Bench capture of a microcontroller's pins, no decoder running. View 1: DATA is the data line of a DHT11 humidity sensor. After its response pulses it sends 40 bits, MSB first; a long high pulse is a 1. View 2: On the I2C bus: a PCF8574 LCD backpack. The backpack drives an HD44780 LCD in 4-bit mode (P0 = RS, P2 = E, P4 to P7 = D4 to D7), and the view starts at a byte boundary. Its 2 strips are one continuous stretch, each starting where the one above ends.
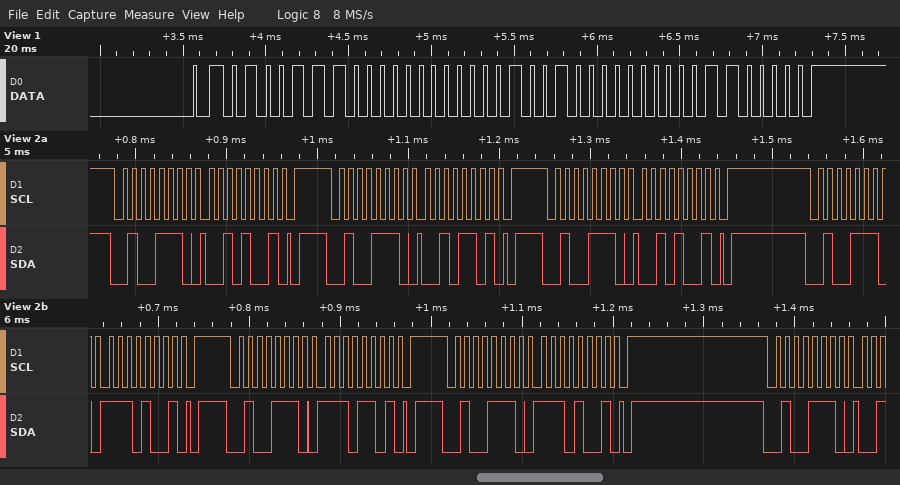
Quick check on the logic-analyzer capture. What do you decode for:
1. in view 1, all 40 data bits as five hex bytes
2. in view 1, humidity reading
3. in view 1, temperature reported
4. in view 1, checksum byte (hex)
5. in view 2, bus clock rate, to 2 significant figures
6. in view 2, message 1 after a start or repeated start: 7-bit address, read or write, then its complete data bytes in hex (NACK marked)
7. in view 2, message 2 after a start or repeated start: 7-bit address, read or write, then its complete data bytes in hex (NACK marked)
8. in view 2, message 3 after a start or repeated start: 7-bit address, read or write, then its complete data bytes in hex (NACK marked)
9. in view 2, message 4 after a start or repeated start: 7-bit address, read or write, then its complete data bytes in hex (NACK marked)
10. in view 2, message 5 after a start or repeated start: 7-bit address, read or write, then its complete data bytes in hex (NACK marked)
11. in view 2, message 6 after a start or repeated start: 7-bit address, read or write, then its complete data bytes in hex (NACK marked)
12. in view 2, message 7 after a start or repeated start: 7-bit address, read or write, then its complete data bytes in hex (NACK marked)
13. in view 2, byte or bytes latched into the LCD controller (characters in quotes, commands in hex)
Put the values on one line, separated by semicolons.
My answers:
4E 00 12 00 60; 78 %; 18.0 °C; 0x60; 100 kHz; 0x27 write: 29; 0x27 write: 2D; 0x27 write: 29; 0x27 write: E9; 0x27 write: ED; 0x27 write: E9; 0x27 write; '.'
